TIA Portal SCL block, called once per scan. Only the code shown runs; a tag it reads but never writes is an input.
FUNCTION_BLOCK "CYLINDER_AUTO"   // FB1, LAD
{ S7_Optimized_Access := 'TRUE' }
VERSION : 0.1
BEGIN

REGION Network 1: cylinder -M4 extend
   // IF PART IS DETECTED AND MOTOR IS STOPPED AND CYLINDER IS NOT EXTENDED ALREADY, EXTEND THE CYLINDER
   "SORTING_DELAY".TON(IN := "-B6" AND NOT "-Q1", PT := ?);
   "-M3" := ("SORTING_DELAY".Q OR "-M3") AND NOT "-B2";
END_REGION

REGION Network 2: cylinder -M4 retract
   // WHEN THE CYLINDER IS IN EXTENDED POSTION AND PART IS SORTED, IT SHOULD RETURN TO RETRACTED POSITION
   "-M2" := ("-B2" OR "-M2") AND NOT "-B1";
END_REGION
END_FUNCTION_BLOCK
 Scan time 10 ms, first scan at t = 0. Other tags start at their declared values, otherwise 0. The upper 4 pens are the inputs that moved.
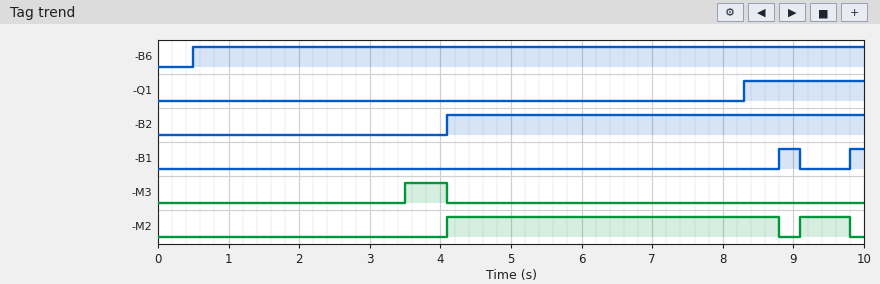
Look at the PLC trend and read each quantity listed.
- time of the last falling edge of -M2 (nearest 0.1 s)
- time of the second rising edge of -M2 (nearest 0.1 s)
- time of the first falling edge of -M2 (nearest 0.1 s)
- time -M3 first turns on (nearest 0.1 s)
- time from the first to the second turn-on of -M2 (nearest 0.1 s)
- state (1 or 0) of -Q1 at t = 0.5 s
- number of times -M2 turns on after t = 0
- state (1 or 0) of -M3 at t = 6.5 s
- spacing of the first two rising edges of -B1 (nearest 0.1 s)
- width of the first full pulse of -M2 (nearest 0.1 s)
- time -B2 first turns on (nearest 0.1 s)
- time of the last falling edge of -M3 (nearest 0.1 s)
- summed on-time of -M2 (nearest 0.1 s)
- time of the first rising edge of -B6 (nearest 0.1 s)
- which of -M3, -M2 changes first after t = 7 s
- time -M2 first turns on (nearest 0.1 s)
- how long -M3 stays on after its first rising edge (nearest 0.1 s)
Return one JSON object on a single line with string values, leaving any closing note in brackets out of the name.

{"time of the last falling edge of -M2": "9.8 s", "time of the second rising edge of -M2": "9.1 s", "time of the first falling edge of -M2": "8.8 s", "time -M3 first turns on": "3.5 s", "time from the first to the second turn-on of -M2": "5.0 s", "state (1 or 0) of -Q1 at t = 0.5 s": "0", "number of times -M2 turns on after t = 0": "2", "state (1 or 0) of -M3 at t = 6.5 s": "0", "spacing of the first two rising edges of -B1": "1.0 s", "width of the first full pulse of -M2": "4.7 s", "time -B2 first turns on": "4.1 s", "time of the last falling edge of -M3": "4.1 s", "summed on-time of -M2": "5.4 s", "time of the first rising edge of -B6": "0.5 s", "which of -M3, -M2 changes first after t = 7 s": "-M2", "time -M2 first turns on": "4.1 s", "how long -M3 stays on after its first rising edge": "0.6 s"}
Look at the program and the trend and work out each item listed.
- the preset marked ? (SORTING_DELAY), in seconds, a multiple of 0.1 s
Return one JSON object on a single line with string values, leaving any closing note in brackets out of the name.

{"the preset marked ? (SORTING_DELAY), in seconds, a multiple of 0.1 s": "3.0 s"}
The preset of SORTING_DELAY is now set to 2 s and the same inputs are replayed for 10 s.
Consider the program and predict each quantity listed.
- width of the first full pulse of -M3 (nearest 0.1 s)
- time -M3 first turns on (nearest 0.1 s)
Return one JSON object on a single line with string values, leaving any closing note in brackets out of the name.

{"width of the first full pulse of -M3": "1.6 s", "time -M3 first turns on": "2.5 s"}
